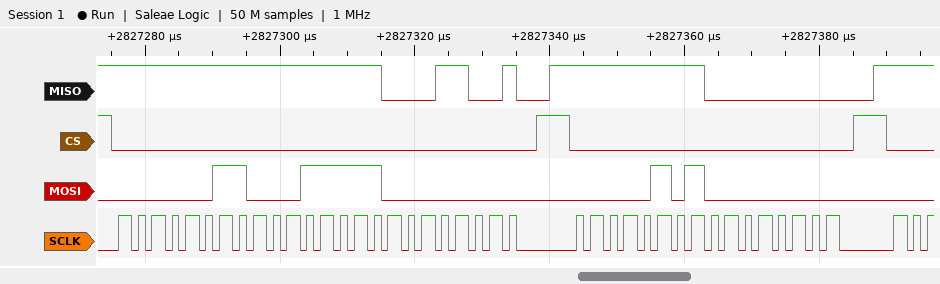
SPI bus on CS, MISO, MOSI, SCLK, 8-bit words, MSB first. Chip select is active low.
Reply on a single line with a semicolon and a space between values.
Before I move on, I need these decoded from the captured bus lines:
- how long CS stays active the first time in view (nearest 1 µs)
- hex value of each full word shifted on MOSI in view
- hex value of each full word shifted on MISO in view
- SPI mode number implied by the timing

63 µs; 03, 1F, 00, 05, 00; FF, FF, 19, FF, 00; 0
